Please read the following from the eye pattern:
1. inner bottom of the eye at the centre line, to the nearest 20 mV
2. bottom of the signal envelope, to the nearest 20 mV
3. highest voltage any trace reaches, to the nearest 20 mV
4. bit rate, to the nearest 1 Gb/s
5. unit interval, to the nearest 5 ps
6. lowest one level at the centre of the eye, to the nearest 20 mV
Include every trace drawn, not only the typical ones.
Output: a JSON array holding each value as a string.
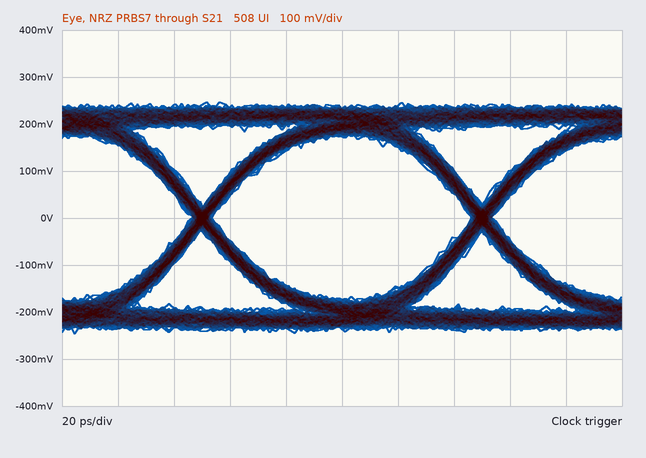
["-180 mV", "-240 mV", "240 mV", "10 Gb/s", "100 ps", "180 mV"]
